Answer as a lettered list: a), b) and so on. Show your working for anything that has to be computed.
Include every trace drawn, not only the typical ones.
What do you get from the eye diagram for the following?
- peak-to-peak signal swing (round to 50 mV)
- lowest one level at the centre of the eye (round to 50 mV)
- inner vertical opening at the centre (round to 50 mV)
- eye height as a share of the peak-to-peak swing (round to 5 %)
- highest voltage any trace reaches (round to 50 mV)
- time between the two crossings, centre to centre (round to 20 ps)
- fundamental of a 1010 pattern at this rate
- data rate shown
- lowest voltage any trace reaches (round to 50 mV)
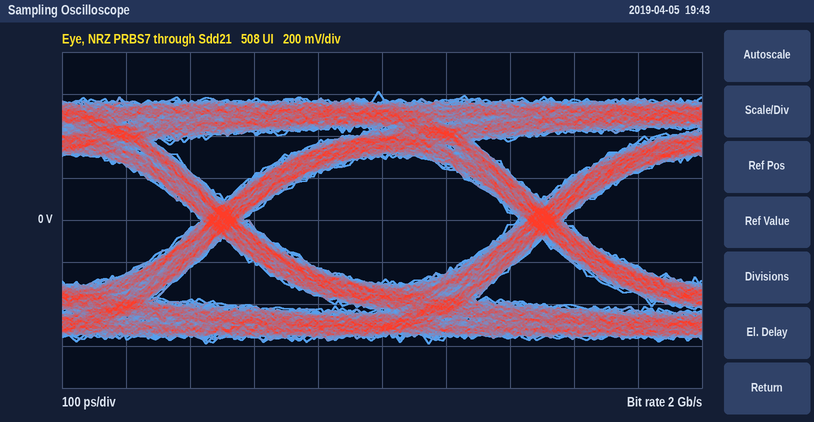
a) 1.20 V
b) 300 mV
c) 600 mV
d) 600 mV / 1.20 V ≈ 50 %
e) 600 mV
f) 500 ps
g) 1 GHz
h) 2 Gb/s
i) -600 mV
